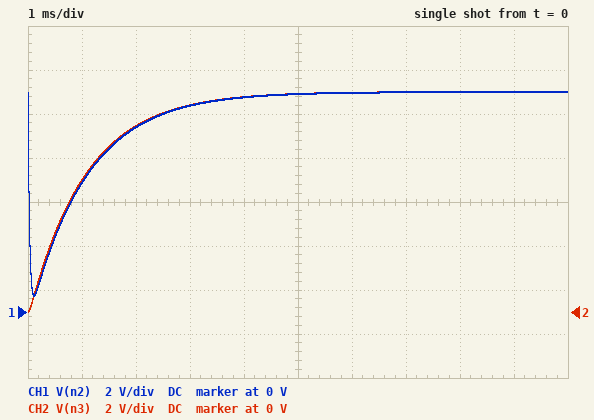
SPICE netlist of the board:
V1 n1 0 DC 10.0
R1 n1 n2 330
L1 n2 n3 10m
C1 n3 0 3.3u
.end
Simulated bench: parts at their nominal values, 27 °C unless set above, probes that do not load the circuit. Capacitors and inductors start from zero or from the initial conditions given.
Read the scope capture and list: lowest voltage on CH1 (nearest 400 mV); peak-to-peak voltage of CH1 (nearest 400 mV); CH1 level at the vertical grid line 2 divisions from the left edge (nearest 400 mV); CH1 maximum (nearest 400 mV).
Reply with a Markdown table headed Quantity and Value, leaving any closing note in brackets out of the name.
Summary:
| Quantity | Value |
|---|---|
| lowest voltage on CH1 | 800 mV |
| peak-to-peak voltage of CH1 | 9.2 V |
| CH1 level at the vertical grid line 2 divisions from the left edge | 8.4 V |
| CH1 maximum | 10.0 V |
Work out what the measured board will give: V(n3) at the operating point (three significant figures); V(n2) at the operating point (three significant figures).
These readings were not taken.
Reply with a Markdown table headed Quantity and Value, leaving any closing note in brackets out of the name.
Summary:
| Quantity | Value |
|---|---|
| V(n3) at the operating point | 10.0 V |
| V(n2) at the operating point | 10.0 V |
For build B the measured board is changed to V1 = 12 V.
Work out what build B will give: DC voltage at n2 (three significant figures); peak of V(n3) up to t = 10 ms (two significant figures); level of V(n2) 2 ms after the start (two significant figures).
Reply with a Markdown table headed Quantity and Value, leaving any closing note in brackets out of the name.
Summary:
| Quantity | Value |
|---|---|
| DC voltage at n2 | 12.0 V |
| peak of V(n3) up to t = 10 ms | 12 V |
| level of V(n2) 2 ms after the start | 10 V |
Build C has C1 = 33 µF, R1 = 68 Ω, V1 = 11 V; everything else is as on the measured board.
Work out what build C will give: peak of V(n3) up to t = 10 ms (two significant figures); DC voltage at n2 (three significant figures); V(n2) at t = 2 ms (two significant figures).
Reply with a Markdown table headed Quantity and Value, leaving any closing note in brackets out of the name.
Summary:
| Quantity | Value |
|---|---|
| peak of V(n3) up to t = 10 ms | 11 V |
| DC voltage at n2 | 11.0 V |
| V(n2) at t = 2 ms | 6.1 V |
